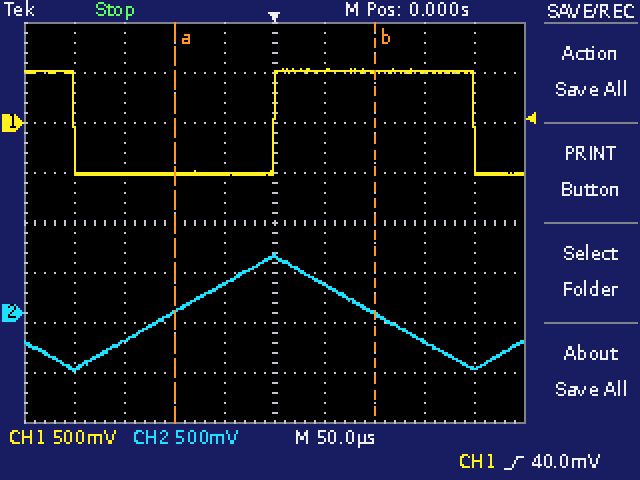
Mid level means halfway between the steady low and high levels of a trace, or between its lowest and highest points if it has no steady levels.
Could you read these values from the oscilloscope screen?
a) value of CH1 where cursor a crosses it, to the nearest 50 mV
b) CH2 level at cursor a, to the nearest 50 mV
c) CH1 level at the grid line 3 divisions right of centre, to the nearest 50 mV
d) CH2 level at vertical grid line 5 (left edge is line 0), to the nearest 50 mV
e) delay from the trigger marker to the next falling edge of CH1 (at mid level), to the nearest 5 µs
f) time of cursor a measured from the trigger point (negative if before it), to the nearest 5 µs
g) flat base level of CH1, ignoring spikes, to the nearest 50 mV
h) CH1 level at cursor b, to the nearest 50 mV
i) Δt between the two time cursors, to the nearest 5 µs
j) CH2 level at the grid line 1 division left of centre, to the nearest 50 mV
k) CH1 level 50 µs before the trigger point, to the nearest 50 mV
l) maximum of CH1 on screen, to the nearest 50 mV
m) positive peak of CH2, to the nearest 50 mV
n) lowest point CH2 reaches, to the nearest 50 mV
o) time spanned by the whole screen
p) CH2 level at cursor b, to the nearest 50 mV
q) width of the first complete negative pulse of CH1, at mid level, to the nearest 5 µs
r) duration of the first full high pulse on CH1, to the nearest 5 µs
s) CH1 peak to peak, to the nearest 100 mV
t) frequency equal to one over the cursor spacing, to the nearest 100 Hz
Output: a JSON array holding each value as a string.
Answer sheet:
["-500 mV", "0 mV", "500 mV", "550 mV", "200 µs", "-100 µs", "-500 mV", "500 mV", "200 µs", "300 mV", "-500 mV", "550 mV", "600 mV", "-600 mV", "500 µs", "0 mV", "200 µs", "200 µs", "1.10 V", "5.0 kHz"]
